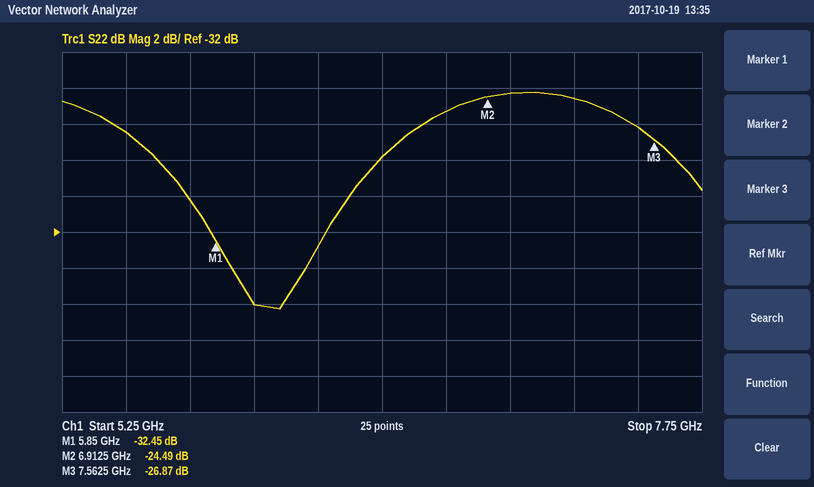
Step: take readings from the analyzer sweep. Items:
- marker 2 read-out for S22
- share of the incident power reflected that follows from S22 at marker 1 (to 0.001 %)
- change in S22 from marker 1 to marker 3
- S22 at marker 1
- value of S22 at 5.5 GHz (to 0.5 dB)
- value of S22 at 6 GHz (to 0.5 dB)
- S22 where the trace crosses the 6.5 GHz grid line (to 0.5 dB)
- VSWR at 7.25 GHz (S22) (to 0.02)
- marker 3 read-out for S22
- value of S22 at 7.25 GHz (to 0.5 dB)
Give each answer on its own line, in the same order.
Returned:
-24.49 dB
0.057 %
5.58 dB
-32.45 dB
-26.5 dB
-36.0 dB
-28.0 dB
1.12
-26.87 dB
-24.5 dB
